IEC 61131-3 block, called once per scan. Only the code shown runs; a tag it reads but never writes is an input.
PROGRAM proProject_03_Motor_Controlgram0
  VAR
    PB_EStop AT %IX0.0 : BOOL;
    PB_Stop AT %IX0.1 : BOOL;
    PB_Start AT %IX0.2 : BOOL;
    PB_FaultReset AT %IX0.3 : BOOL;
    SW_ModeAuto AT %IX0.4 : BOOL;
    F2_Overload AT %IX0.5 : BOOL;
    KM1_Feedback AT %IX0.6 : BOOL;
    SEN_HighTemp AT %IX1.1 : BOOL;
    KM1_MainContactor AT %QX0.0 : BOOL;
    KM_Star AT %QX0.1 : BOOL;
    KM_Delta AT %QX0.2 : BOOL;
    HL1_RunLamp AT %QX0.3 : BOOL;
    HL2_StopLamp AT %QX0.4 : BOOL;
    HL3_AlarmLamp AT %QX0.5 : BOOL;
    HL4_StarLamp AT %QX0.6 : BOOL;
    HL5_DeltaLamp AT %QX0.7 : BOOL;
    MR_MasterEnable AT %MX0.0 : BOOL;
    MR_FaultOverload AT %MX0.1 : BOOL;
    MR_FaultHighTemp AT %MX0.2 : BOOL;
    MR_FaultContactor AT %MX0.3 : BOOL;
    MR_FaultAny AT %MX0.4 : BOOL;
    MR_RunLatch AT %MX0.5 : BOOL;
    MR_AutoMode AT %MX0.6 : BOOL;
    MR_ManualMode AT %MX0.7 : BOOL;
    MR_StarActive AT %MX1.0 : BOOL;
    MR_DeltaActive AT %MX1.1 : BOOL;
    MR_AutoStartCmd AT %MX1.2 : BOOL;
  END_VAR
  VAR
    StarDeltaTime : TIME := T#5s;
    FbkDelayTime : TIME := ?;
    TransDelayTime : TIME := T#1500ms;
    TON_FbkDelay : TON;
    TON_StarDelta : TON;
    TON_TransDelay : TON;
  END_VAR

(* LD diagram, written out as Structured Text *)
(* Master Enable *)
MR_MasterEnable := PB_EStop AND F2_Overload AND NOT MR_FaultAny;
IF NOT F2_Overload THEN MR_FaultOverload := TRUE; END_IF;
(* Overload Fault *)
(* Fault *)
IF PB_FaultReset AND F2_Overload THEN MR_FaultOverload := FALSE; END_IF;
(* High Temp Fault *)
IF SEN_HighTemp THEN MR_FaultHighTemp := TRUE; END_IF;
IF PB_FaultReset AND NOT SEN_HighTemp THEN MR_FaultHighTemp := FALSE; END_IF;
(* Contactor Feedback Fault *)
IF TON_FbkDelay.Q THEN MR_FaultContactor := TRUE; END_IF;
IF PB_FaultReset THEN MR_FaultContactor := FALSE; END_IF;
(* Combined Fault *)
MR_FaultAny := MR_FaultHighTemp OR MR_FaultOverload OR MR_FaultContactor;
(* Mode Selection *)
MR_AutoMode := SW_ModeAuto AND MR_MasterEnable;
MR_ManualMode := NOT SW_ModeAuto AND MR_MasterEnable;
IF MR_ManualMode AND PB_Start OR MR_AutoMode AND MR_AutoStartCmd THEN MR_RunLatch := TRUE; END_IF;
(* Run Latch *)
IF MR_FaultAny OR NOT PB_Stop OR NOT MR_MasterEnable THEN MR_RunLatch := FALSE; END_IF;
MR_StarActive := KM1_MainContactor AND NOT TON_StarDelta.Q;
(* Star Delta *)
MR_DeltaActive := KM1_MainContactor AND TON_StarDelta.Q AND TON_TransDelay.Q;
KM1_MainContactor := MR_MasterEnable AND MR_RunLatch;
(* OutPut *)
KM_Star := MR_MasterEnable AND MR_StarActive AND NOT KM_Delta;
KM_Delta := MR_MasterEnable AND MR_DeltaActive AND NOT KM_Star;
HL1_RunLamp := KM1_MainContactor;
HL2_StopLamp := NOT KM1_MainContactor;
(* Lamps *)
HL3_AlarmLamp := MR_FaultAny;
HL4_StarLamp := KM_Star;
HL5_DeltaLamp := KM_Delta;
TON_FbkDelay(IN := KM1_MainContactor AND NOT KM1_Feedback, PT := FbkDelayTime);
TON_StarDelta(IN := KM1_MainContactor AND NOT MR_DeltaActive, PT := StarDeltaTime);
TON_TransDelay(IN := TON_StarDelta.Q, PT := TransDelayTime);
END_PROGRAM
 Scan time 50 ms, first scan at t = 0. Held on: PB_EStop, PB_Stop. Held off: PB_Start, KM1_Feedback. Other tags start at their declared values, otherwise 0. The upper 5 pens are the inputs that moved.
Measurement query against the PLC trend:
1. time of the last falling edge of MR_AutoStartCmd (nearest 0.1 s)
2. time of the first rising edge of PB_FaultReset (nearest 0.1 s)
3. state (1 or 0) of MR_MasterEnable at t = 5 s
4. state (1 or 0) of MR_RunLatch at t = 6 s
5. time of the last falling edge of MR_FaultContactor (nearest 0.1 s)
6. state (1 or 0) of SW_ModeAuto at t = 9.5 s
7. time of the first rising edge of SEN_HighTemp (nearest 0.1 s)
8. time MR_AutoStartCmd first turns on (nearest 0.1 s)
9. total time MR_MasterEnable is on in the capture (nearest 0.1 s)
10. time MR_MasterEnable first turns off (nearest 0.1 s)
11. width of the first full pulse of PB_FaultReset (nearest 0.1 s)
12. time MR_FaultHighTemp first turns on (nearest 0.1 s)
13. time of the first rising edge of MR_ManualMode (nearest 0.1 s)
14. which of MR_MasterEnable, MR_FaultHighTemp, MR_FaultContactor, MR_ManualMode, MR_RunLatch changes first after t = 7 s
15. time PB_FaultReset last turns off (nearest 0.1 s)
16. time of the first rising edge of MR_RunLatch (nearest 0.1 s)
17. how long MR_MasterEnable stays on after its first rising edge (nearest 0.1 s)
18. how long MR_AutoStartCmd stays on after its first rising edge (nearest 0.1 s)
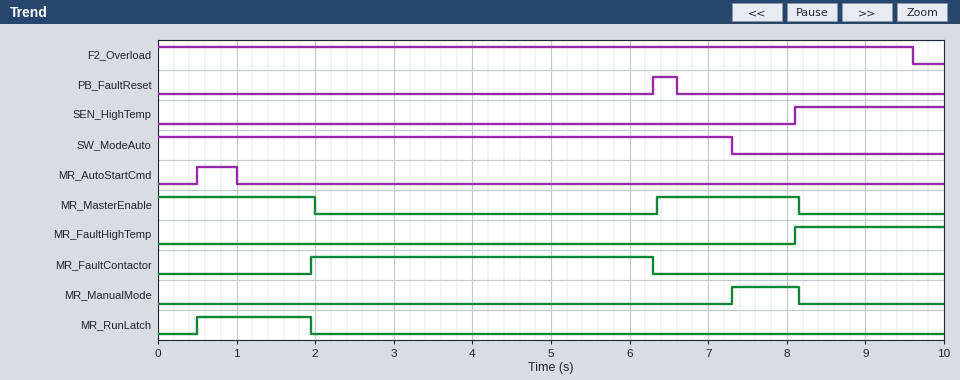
1.0 s
6.3 s
0
0
6.3 s
0
8.1 s
0.5 s
3.8 s
2.0 s
0.3 s
8.1 s
7.3 s
MR_ManualMode
6.6 s
0.5 s
1.8 s
0.5 s
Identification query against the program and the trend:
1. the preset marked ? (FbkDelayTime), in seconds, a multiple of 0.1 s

1.4 s
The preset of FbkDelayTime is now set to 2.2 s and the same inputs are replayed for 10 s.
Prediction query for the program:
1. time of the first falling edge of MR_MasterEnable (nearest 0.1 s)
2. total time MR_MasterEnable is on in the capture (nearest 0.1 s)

2.8 s
4.6 s
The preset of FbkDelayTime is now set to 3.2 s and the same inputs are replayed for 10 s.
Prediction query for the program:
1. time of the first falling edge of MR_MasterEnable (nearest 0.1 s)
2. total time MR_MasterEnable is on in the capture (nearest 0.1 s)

3.8 s
5.6 s
